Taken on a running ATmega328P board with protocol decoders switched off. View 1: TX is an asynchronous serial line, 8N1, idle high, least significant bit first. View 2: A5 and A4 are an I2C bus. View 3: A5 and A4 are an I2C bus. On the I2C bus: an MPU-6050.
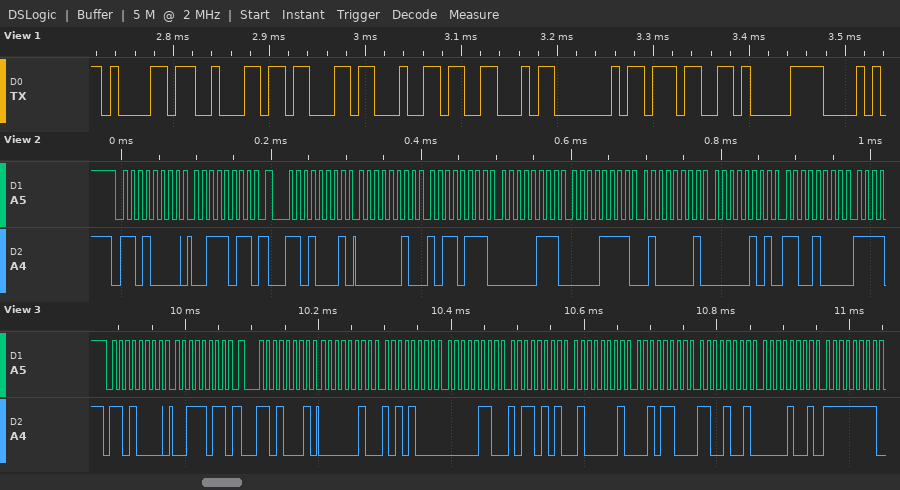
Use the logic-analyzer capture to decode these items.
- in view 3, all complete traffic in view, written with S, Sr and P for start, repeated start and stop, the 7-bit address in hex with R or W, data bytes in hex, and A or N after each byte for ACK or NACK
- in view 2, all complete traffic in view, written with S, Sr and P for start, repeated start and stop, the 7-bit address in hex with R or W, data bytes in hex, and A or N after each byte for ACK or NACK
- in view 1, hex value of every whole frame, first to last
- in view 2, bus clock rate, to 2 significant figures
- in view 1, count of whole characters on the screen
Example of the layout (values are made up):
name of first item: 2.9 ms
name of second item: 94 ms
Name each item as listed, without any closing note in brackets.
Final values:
in view 3, all complete traffic in view, written with S, Sr and P for start, repeated start and stop, the 7-bit address in hex with R or W, data bytes in hex, and A or N after each byte for ACK or NACK: S 68W A 3B A Sr 68R A 02 A A8 A 06 A B5 A 41 A 2C A C9 A 09 A FF A
in view 2, all complete traffic in view, written with S, Sr and P for start, repeated start and stop, the 7-bit address in hex with R or W, data bytes in hex, and A or N after each byte for ACK or NACK: S 68W A 3B A Sr 68R A 02 A B7 A 07 A 0F A 41 A 05 A C8 A
in view 1, hex value of every whole frame, first to last: 61 62 63 64 46 40 37 C1
in view 2, bus clock rate, to 2 significant figures: 100 kHz
in view 1, count of whole characters on the screen: 8
